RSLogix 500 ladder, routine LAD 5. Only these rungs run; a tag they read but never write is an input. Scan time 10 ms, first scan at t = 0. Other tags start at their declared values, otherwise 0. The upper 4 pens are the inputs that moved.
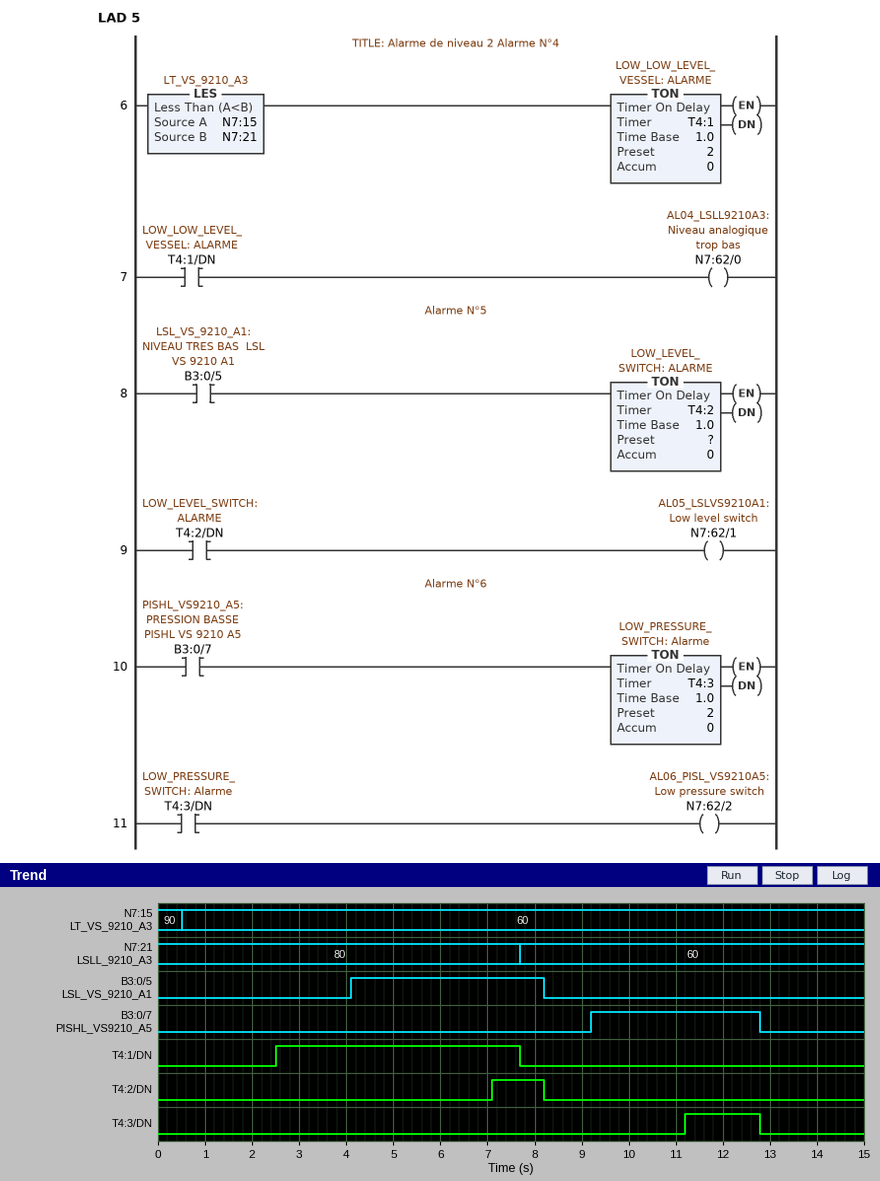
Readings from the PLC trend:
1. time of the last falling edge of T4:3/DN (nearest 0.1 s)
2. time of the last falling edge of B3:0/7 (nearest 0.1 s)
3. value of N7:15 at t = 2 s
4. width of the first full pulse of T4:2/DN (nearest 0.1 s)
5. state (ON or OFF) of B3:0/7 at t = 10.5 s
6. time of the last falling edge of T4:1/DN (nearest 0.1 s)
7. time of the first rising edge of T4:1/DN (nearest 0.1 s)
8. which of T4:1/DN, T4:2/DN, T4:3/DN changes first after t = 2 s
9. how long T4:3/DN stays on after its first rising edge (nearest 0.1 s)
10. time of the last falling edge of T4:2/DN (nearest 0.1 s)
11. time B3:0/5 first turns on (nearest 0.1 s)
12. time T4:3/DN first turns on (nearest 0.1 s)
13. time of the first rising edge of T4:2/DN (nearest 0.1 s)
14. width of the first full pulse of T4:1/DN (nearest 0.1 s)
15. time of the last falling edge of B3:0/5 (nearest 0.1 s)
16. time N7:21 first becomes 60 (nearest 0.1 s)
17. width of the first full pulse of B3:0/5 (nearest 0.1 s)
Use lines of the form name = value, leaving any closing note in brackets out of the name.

time of the last falling edge of T4:3/DN = 12.8 s
time of the last falling edge of B3:0/7 = 12.8 s
value of N7:15 at t = 2 s = 60
width of the first full pulse of T4:2/DN = 1.1 s
state (ON or OFF) of B3:0/7 at t = 10.5 s = ON
time of the last falling edge of T4:1/DN = 7.7 s
time of the first rising edge of T4:1/DN = 2.5 s
which of T4:1/DN, T4:2/DN, T4:3/DN changes first after t = 2 s = T4:1/DN
how long T4:3/DN stays on after its first rising edge = 1.6 s
time of the last falling edge of T4:2/DN = 8.2 s
time B3:0/5 first turns on = 4.1 s
time T4:3/DN first turns on = 11.2 s
time of the first rising edge of T4:2/DN = 7.1 s
width of the first full pulse of T4:1/DN = 5.2 s
time of the last falling edge of B3:0/5 = 8.2 s
time N7:21 first becomes 60 = 7.7 s
width of the first full pulse of B3:0/5 = 4.1 s
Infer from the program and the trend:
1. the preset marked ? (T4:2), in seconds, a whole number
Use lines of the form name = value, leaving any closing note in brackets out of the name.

the preset marked ? (T4:2), in seconds, a whole number = 3 s
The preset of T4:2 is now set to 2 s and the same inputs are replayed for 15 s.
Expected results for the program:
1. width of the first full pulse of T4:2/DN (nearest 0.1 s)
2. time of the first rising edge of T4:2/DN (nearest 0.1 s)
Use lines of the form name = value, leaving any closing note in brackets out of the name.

width of the first full pulse of T4:2/DN = 2.1 s
time of the first rising edge of T4:2/DN = 6.1 s
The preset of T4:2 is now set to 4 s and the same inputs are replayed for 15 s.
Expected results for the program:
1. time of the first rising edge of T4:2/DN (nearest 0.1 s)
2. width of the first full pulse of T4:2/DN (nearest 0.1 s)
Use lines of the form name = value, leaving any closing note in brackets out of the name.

time of the first rising edge of T4:2/DN = 8.1 s
width of the first full pulse of T4:2/DN = 0.1 s
